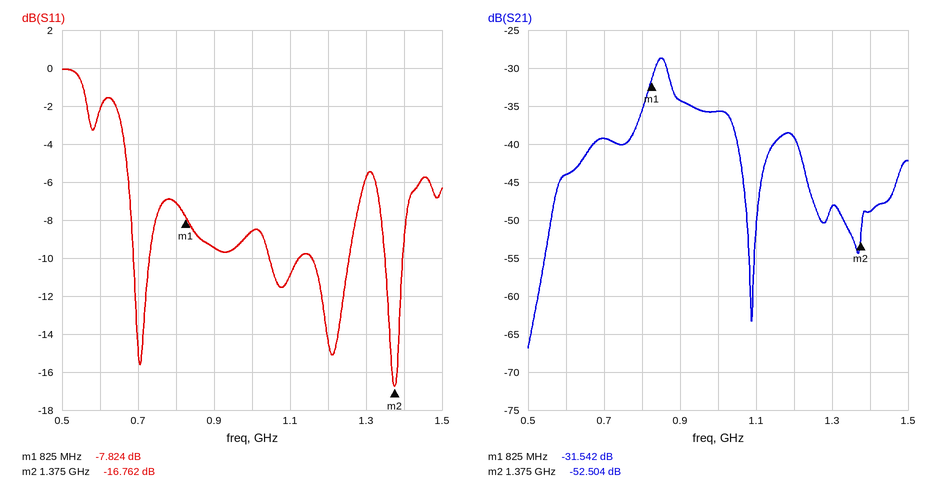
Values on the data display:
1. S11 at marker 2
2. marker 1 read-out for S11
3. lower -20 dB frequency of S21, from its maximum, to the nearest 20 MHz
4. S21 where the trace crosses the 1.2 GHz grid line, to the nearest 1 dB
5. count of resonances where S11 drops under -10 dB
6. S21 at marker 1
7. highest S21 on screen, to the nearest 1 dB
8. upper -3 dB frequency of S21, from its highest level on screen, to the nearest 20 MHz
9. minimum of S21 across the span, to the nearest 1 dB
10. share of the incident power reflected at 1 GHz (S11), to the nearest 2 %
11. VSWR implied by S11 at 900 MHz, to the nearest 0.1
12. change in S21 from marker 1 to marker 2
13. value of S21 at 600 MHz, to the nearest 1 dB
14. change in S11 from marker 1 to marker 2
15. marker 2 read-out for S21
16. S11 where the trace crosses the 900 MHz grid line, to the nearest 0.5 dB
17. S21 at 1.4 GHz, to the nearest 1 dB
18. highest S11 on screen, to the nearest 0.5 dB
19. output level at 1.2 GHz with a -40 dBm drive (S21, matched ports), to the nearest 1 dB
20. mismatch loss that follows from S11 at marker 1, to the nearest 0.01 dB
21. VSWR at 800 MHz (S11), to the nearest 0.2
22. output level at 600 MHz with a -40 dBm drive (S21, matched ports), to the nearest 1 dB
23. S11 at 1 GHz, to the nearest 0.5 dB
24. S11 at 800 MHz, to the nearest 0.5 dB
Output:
-16.762 dB
-7.824 dB
560 MHz
-39 dB
3
-31.542 dB
-29 dB
880 MHz
-67 dB
14 %
2.0
-20.962 dB
-44 dB
-8.938 dB
-52.504 dB
-9.5 dB
-49 dB
0.0 dB
-79 dBm
0.78 dB
2.6
-84 dBm
-8.5 dB
-7.0 dB
